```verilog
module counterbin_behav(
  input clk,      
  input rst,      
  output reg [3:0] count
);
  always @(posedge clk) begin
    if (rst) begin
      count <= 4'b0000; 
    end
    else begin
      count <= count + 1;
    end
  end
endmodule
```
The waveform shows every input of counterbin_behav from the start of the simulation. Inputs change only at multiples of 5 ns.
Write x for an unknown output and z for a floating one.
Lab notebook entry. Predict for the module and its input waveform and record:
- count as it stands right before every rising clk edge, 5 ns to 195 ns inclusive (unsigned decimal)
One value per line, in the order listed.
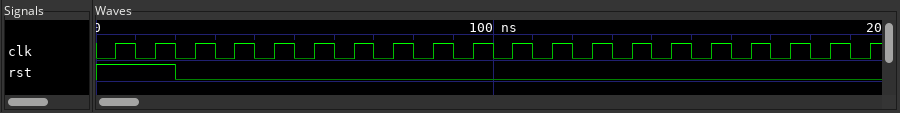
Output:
x, 0, 0, 1, 2, 3, 4, 5, 6, 7, 8, 9, 10, 11, 12, 13, 14, 15, 0, 1
